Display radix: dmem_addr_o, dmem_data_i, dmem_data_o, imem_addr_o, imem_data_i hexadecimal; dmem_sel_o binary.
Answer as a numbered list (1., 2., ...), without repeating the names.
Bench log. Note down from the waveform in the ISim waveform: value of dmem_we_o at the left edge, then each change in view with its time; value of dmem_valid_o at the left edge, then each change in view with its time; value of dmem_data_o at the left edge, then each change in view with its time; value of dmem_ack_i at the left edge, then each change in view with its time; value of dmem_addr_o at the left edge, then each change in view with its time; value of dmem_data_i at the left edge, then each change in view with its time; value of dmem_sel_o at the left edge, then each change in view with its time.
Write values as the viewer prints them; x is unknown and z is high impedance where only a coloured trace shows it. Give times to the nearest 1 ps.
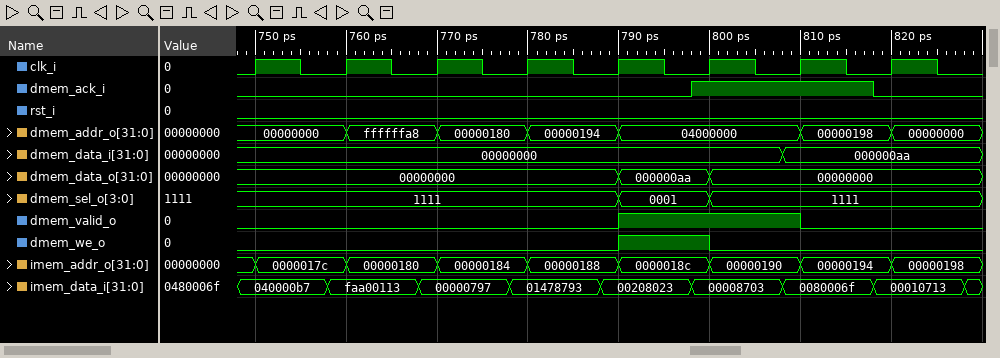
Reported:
1. 0, 1 at 790 ps, 0 at 800 ps
2. 0, 1 at 790 ps, 0 at 810 ps
3. 00000000, 000000aa at 790 ps, 00000000 at 800 ps
4. 0, 1 at 798 ps, 0 at 818 ps
5. 00000000, ffffffa8 at 760 ps, 00000180 at 770 ps, 00000194 at 780 ps, 04000000 at 790 ps, 00000198 at 810 ps, 00000000 at 820 ps
6. 00000000, 000000aa at 808 ps
7. 1111, 0001 at 790 ps, 1111 at 800 ps
